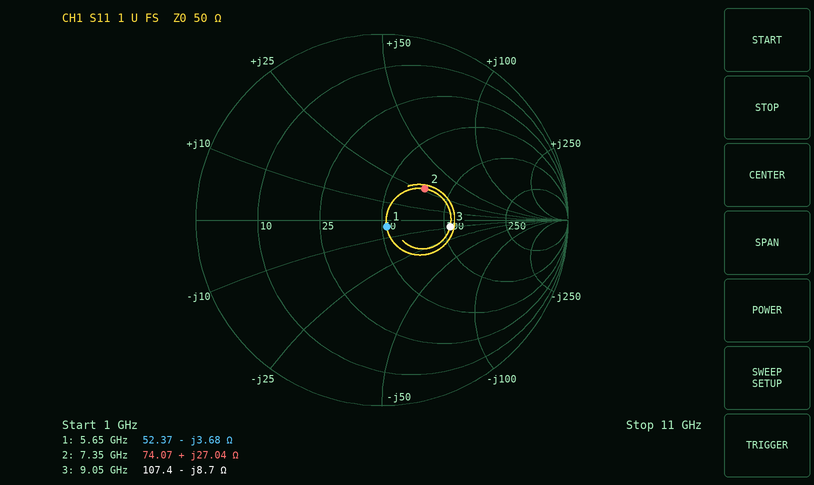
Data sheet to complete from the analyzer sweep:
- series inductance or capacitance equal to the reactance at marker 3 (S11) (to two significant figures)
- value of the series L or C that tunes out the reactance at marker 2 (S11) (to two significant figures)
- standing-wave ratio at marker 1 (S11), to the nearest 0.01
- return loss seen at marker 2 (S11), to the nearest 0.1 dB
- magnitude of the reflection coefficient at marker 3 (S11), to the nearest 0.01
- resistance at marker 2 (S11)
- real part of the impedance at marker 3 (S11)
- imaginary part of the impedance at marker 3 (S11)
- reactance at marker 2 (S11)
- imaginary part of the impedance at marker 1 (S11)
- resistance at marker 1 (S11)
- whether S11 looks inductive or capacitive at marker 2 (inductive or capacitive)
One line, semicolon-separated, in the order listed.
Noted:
2.0 pF; 800 fF; 1.09; 10.9 dB; 0.37; 74.07 Ω; 107.4 Ω; -8.7 Ω; +27.04 Ω; -3.68 Ω; 52.37 Ω; inductive
